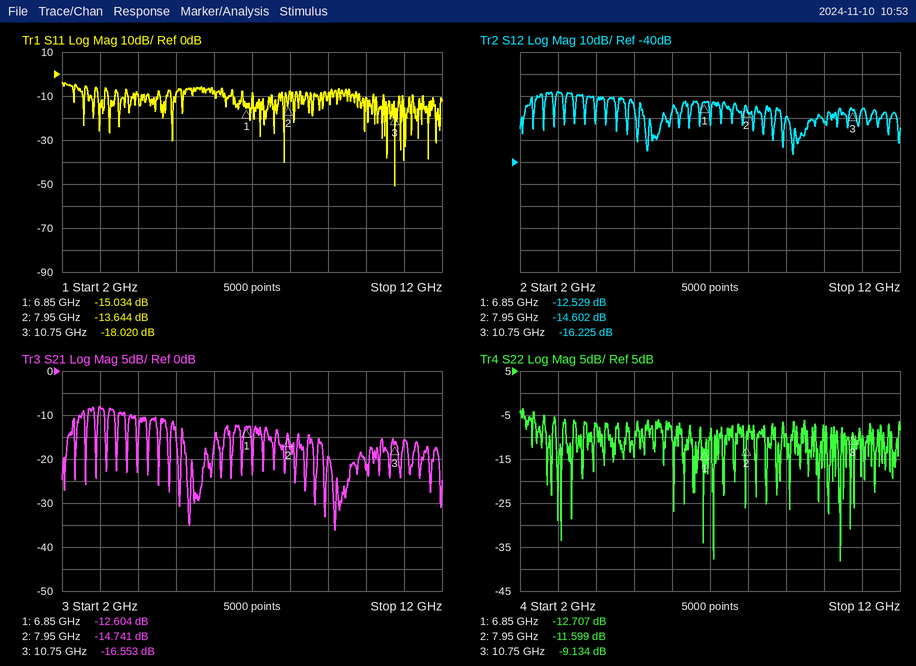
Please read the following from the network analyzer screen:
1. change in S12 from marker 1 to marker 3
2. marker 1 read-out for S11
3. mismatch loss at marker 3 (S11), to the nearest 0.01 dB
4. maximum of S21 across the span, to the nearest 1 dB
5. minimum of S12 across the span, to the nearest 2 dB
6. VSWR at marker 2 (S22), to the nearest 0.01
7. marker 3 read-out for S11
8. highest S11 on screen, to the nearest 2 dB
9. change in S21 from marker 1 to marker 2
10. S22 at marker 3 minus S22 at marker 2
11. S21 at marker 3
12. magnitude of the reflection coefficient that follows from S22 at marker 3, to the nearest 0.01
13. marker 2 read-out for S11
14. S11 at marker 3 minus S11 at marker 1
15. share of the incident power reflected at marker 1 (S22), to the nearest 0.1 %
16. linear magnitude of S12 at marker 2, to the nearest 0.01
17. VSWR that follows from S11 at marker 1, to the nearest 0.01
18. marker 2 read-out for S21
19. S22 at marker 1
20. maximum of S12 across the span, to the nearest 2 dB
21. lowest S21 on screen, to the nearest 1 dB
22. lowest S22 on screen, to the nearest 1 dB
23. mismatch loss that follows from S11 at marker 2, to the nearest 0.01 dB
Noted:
-3.696 dB
-15.034 dB
0.07 dB
-8 dB
-36 dB
1.71
-18.020 dB
-4 dB
-2.137 dB
2.465 dB
-16.553 dB
0.35
-13.644 dB
-2.986 dB
5.4 %
0.19
1.43
-14.741 dB
-12.707 dB
-8 dB
-36 dB
-38 dB
0.19 dB
